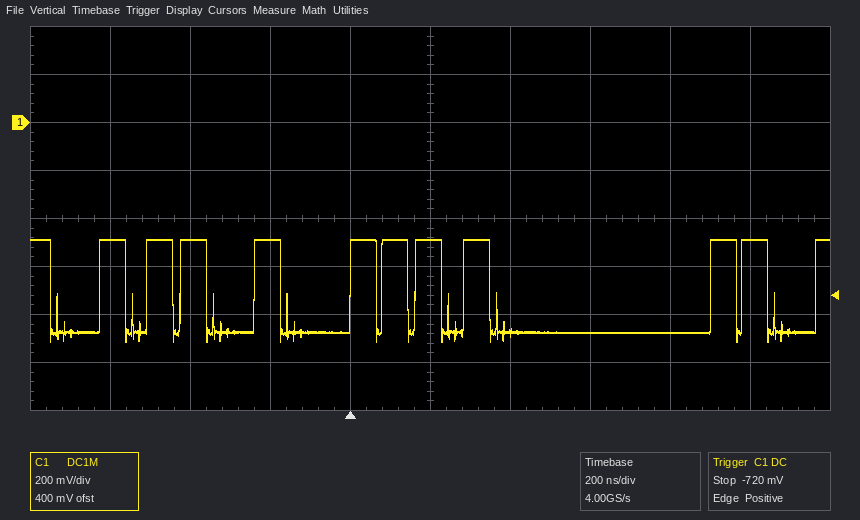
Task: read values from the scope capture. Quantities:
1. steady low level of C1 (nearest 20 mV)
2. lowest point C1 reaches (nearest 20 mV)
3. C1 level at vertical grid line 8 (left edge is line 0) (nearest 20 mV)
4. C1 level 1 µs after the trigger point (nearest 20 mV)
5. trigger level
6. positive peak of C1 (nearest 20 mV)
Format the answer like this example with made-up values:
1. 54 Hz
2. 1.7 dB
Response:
1. -880 mV
2. -920 mV
3. -880 mV
4. -480 mV
5. -720 mV
6. -480 mV
